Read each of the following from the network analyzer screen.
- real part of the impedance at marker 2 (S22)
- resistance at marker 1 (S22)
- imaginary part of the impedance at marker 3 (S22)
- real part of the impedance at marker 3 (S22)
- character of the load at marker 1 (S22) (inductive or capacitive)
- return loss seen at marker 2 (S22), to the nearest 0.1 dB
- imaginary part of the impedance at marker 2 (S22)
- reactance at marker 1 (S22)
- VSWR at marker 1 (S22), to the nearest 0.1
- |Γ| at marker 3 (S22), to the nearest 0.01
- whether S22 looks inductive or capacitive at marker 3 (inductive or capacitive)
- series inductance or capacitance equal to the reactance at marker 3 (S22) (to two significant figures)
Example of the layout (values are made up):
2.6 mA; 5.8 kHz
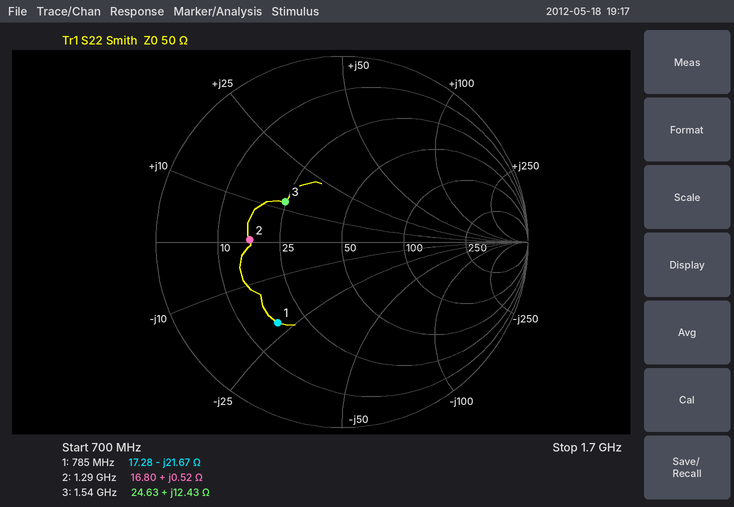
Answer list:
16.80 Ω; 17.28 Ω; +12.43 Ω; 24.63 Ω; capacitive; 6.1 dB; +0.52 Ω; -21.67 Ω; 3.5; 0.37; inductive; 1.3 nH
